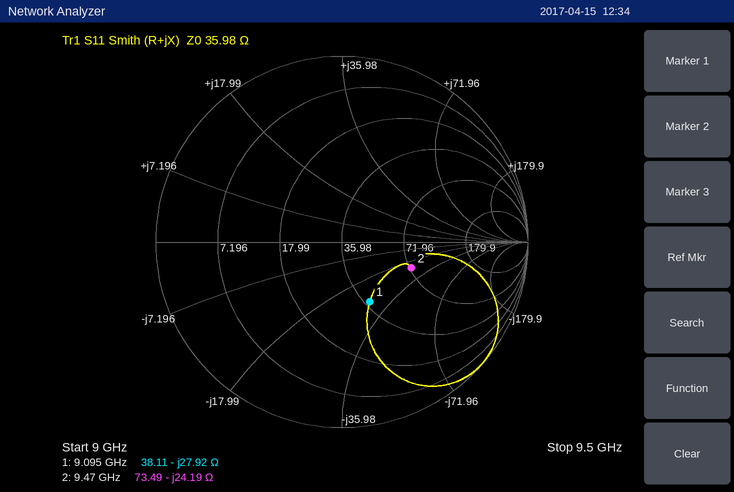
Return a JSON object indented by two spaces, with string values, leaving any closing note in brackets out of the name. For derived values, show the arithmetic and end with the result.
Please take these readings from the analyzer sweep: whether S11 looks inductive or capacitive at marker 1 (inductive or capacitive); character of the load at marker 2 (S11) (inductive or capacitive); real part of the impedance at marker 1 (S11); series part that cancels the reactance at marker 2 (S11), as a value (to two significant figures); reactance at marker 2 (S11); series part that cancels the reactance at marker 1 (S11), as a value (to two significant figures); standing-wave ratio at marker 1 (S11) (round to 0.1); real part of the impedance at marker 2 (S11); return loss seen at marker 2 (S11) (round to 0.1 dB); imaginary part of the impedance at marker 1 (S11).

{
  "whether S11 looks inductive or capacitive at marker 1": "capacitive",
  "character of the load at marker 2 (S11)": "capacitive",
  "real part of the impedance at marker 1": "38.11 Ω",
  "series part that cancels the reactance at marker 2 (S11), as a value": "L = 24.19 Ω/(2π × 9.47 GHz) ≈ 407 pH, so 410 pH to two significant figures",
  "reactance at marker 2": "-24.19 Ω",
  "series part that cancels the reactance at marker 1 (S11), as a value": "L = 27.92 Ω/(2π × 9.095 GHz) ≈ 489 pH, so 490 pH to two significant figures",
  "standing-wave ratio at marker 1 (S11)": "2.1",
  "real part of the impedance at marker 2": "73.49 Ω",
  "return loss seen at marker 2 (S11)": "8.0 dB",
  "imaginary part of the impedance at marker 1": "-27.92 Ω"
}
